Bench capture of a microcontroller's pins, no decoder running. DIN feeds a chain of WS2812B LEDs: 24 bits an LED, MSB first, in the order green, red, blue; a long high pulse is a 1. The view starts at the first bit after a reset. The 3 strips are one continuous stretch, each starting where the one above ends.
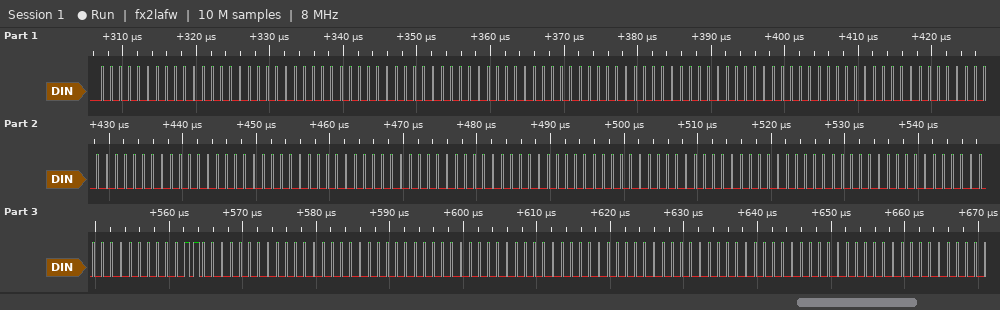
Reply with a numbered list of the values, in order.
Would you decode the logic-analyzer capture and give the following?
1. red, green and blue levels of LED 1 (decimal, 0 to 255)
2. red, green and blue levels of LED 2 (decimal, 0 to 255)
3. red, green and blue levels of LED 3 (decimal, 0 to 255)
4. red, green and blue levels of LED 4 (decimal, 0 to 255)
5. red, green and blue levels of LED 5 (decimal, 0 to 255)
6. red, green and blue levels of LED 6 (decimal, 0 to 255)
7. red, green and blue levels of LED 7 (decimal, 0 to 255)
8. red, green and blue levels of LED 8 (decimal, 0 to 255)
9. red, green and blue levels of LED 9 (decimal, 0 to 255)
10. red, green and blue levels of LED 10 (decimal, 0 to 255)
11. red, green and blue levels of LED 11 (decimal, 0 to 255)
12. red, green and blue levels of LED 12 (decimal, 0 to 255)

1. 0, 0, 0
2. 0, 0, 0
3. 0, 0, 0
4. 0, 0, 0
5. 0, 0, 0
6. 0, 0, 0
7. 0, 0, 0
8. 0, 0, 0
9. 12, 0, 0
10. 0, 0, 0
11. 0, 0, 0
12. 0, 0, 0
